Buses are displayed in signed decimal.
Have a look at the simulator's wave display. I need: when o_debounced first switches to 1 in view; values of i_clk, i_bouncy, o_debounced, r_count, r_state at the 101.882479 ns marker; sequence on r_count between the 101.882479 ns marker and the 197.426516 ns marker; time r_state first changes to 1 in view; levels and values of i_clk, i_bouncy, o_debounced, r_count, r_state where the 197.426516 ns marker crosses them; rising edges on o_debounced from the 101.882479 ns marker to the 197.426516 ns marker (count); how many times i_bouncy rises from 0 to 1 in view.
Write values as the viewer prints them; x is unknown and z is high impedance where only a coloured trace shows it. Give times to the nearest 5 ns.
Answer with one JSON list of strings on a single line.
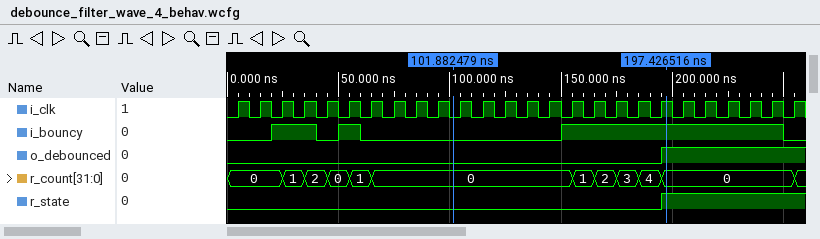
["195 ns", "i_clk=0, i_bouncy=0, o_debounced=0, r_count=0, r_state=0", "0, 1, 2, 3, 4, 0", "195 ns", "i_clk=1, i_bouncy=1, o_debounced=1, r_count=0, r_state=1", "1", "3"]
